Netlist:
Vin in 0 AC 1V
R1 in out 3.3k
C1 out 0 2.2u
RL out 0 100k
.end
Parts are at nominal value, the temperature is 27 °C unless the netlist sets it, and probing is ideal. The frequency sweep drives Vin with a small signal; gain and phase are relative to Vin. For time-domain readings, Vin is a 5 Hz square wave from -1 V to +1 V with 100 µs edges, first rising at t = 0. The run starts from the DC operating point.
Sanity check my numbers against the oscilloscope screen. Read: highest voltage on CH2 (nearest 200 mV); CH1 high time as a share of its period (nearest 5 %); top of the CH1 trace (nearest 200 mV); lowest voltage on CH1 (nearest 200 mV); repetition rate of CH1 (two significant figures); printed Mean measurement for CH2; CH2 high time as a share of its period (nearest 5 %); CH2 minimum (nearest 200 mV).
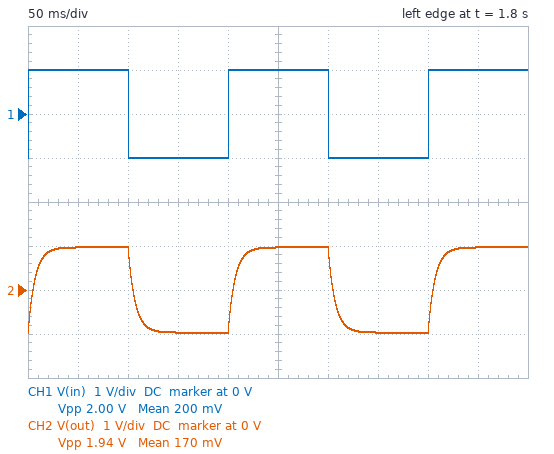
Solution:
1.0 V
50 %
1.0 V
-1.0 V
5.0 Hz
170 mV
50 %
-1.0 V
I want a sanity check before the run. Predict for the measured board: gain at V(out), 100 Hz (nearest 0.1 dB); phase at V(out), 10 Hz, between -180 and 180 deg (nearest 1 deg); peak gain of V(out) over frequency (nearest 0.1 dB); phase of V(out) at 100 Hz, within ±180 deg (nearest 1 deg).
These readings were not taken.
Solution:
-13.4 dB
-24 deg
-0.3 dB
-77 deg
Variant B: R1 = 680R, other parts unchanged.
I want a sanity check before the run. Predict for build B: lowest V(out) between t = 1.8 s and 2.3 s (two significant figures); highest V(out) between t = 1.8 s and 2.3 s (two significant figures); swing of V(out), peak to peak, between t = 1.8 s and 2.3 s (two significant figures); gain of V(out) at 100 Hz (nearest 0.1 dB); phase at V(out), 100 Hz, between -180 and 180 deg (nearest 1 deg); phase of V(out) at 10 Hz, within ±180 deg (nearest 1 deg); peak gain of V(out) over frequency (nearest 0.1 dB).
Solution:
-990 mV
990 mV
2.0 V
-2.8 dB
-43 deg
-5 deg
-0.1 dB
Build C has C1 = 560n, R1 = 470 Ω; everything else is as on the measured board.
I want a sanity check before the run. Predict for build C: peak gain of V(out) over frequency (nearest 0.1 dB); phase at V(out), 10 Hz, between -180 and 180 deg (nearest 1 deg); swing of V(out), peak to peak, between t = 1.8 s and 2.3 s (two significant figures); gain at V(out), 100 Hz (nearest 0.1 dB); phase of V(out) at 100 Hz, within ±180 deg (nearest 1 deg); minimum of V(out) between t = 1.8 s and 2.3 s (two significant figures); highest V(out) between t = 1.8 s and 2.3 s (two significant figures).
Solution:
0 dB
-1 deg
2.0 V
-0.2 dB
-9 deg
-1.0 V
1.0 V
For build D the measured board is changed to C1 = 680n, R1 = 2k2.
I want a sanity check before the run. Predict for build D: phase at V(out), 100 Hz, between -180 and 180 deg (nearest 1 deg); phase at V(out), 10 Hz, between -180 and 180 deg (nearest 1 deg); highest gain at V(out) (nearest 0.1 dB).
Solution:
-43 deg
-5 deg
-0.2 dB
